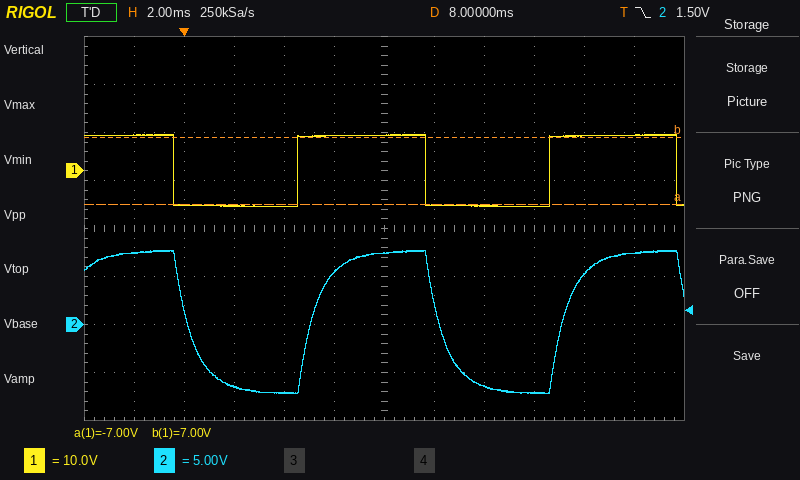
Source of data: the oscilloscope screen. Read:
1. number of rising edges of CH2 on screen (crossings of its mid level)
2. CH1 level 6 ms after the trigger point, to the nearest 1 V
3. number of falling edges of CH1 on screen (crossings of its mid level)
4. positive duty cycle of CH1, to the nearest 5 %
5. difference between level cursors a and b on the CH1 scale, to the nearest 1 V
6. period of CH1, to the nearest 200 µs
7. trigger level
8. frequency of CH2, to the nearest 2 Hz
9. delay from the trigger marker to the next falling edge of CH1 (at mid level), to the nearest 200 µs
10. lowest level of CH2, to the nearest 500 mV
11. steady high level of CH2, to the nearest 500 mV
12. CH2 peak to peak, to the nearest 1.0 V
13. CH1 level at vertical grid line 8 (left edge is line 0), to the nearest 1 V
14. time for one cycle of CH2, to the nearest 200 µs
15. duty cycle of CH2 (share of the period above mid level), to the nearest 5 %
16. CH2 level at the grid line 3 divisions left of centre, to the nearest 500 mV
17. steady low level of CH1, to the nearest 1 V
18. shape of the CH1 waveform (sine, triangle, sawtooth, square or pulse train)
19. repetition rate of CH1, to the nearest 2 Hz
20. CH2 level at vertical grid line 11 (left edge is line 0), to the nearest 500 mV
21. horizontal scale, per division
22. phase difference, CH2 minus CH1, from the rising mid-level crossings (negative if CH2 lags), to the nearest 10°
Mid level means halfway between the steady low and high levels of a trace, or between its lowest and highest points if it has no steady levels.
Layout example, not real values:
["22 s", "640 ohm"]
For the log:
["2", "7 V", "3", "50 %", "14 V", "10.0 ms", "1.50 V", "100 Hz", "9.6 ms", "-7.0 V", "7.5 V", "15.0 V", "-7 V", "10.0 ms", "50 %", "-6.5 V", "-7 V", "square", "100 Hz", "7.5 V", "2 ms", "-20°"]
